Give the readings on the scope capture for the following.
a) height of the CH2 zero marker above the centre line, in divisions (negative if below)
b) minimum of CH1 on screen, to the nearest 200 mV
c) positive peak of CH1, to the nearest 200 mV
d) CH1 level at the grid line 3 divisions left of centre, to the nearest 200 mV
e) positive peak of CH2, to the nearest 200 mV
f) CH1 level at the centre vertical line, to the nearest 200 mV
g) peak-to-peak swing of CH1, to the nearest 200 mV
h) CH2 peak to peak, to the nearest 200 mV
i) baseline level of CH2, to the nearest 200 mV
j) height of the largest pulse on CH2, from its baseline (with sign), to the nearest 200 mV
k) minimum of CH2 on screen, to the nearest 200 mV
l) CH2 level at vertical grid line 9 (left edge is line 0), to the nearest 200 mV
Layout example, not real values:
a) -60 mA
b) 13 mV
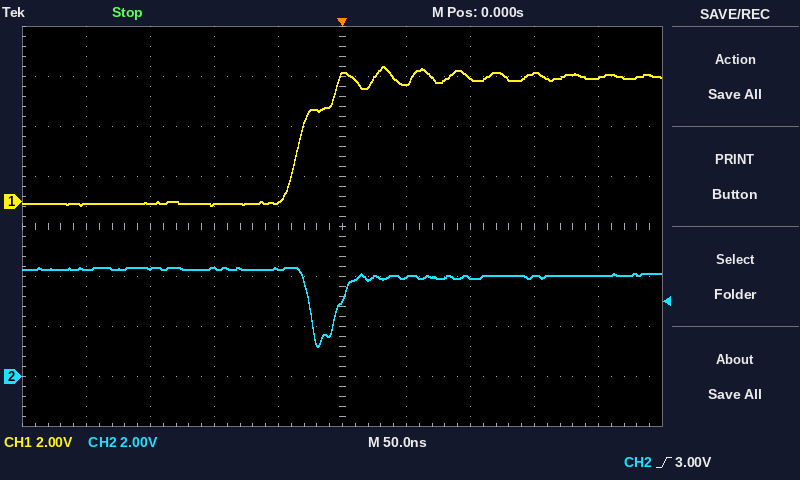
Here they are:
a) -3.0 div
b) -200 mV
c) 5.4 V
d) 0.0 V
e) 4.4 V
f) 5.0 V
g) 5.6 V
h) 3.2 V
i) 4.0 V
j) -2.8 V
k) 1.2 V
l) 4.0 V
